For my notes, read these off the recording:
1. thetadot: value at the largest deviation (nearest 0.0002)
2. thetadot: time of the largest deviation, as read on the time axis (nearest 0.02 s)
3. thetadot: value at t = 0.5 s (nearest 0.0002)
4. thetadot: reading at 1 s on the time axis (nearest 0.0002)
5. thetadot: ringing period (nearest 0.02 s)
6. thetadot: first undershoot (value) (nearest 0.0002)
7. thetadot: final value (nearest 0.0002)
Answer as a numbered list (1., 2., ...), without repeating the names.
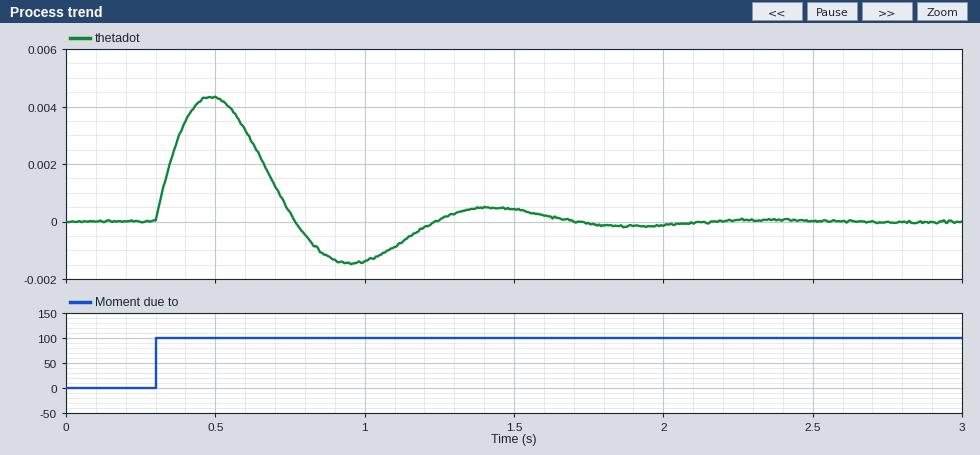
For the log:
1. 0.0044
2. 0.48 s
3. 0.0044
4. -0.0014
5. 0.94 s
6. -0.0014
7. 0.0000
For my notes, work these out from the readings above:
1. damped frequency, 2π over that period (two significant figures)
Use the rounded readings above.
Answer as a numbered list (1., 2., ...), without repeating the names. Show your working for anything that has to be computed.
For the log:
1. 2π / 0.94 = 6.7 rad/s
